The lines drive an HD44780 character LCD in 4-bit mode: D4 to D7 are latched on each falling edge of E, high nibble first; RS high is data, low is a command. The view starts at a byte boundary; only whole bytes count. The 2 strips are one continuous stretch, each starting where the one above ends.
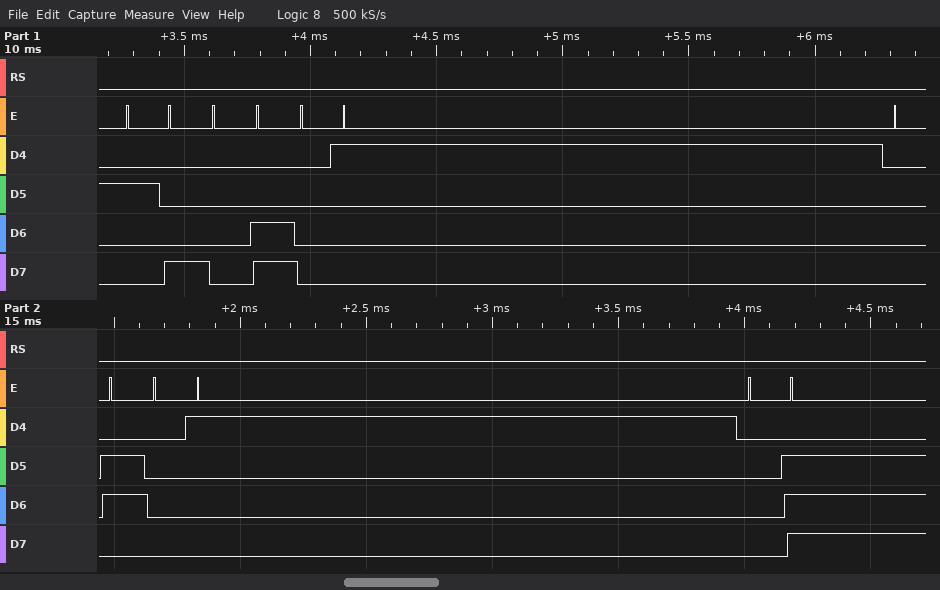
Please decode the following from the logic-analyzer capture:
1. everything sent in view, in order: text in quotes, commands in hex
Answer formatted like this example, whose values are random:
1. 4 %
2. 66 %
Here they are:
1. 0x28 0x0C 0x01 0x06 0x01 0x0E
